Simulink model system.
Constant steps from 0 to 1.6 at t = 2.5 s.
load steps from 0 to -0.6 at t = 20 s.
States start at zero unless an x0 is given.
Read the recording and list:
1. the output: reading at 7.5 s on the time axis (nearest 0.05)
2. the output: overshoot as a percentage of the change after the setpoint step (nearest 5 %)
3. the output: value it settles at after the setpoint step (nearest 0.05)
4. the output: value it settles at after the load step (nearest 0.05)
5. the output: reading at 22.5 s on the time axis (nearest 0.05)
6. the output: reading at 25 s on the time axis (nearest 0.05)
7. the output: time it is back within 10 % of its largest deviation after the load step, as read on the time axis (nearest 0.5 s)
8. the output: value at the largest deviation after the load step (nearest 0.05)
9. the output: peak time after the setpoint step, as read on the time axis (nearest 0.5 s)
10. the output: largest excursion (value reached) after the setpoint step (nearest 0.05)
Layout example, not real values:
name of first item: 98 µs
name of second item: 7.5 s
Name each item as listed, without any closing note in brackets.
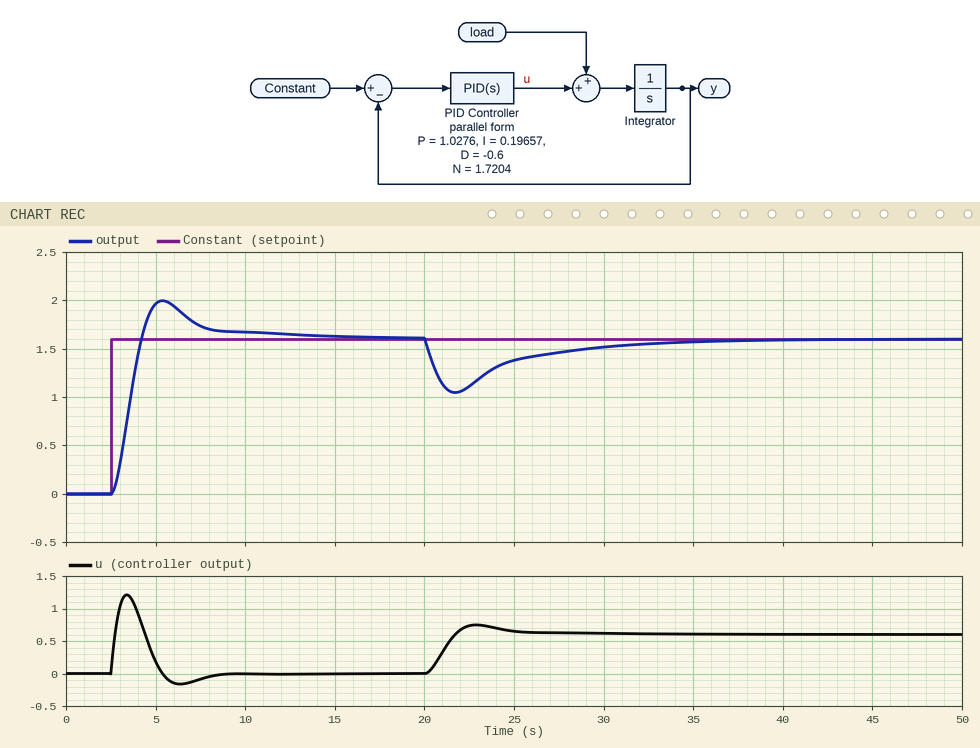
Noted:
the output: reading at 7.5 s on the time axis: 1.75
the output: overshoot as a percentage of the change after the setpoint step: 25 %
the output: value it settles at after the setpoint step: 1.60
the output: value it settles at after the load step: 1.60
the output: reading at 22.5 s on the time axis: 1.10
the output: reading at 25 s on the time axis: 1.40
the output: time it is back within 10 % of its largest deviation after the load step, as read on the time axis: 32.0 s
the output: value at the largest deviation after the load step: 1.05
the output: peak time after the setpoint step, as read on the time axis: 5.5 s
the output: largest excursion (value reached) after the setpoint step: 2.00
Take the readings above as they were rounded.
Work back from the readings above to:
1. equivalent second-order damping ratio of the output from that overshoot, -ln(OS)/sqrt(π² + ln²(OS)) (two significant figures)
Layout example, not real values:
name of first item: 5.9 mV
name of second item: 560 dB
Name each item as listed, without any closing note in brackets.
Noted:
equivalent second-order damping ratio of the output from that overshoot, -ln(OS)/sqrt(π² + ln²(OS)): 0.40
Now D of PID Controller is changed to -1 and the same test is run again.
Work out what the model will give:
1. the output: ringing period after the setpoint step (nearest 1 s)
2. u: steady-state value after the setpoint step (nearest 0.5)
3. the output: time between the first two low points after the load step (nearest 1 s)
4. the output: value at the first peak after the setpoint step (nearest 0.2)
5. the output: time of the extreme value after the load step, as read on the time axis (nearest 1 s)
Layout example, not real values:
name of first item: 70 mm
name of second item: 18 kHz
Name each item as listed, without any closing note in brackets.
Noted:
the output: ringing period after the setpoint step: 5 s
u: steady-state value after the setpoint step: 0.0
the output: time between the first two low points after the load step: 5 s
the output: value at the first peak after the setpoint step: 2.4
the output: time of the extreme value after the load step, as read on the time axis: 22 s
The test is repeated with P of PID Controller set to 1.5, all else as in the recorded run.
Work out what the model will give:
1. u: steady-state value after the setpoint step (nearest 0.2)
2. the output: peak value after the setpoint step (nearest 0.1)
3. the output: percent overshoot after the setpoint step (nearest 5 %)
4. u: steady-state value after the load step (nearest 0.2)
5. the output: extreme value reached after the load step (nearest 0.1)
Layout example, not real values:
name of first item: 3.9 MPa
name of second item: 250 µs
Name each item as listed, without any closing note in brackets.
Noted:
u: steady-state value after the setpoint step: 0.0
the output: peak value after the setpoint step: 1.8
the output: percent overshoot after the setpoint step: 15 %
u: steady-state value after the load step: 0.6
the output: extreme value reached after the load step: 1.2
